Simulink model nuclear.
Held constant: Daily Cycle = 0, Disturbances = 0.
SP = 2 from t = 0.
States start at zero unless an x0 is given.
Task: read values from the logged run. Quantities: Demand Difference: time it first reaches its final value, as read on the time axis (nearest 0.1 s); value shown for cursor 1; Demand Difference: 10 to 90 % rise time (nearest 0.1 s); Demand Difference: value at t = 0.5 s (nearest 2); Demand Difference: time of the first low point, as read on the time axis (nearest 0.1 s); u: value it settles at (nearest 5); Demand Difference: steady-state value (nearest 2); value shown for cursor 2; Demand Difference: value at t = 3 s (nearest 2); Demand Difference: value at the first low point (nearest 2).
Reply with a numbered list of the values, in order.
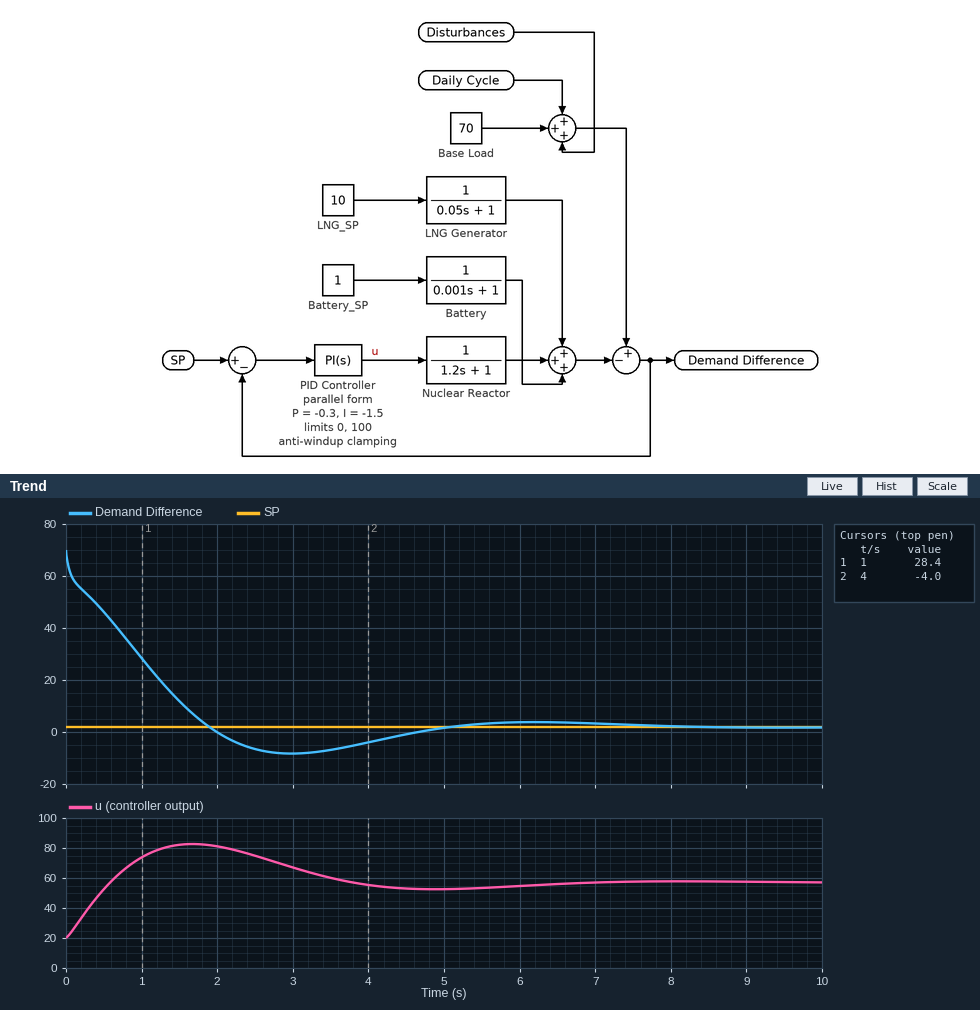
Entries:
1. 1.9 s
2. 28.4
3. 1.6 s
4. 46
5. 3.0 s
6. 55
7. 2
8. -4.0
9. -8
10. -8
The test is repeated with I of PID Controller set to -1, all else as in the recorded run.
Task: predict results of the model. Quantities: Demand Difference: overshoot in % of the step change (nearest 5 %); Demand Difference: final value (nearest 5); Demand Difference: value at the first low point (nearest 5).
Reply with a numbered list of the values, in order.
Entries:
1. 10 %
2. 0
3. -5
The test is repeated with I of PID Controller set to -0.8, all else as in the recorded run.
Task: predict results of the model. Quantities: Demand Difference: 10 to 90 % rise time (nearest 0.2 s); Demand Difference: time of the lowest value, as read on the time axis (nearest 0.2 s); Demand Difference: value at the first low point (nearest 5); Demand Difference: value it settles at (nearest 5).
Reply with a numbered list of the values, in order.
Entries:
1. 2.6 s
2. 4.6 s
3. 0
4. 0
